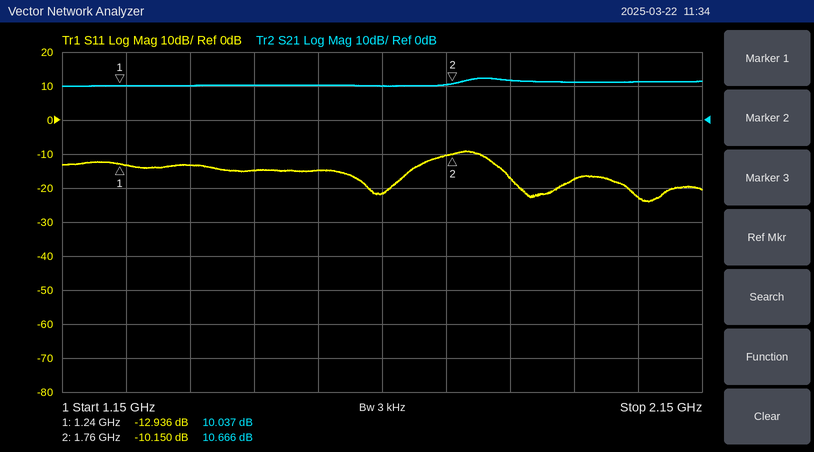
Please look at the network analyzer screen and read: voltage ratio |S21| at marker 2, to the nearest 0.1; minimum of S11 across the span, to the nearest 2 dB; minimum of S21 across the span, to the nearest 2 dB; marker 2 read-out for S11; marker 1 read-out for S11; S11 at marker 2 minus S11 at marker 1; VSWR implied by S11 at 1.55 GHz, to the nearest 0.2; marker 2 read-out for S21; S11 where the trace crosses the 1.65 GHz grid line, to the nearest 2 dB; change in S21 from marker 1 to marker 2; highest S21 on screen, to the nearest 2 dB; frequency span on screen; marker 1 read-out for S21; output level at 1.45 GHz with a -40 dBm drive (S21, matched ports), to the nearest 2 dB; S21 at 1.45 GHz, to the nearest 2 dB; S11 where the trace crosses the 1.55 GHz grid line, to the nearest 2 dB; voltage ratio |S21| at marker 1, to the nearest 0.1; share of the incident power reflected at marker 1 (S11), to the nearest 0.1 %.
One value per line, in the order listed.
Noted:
3.4
-24 dB
10 dB
-10.150 dB
-12.936 dB
2.786 dB
1.4
10.666 dB
-22 dB
0.629 dB
12 dB
1 GHz
10.037 dB
-30 dBm
10 dB
-14 dB
3.2
5.1 %
